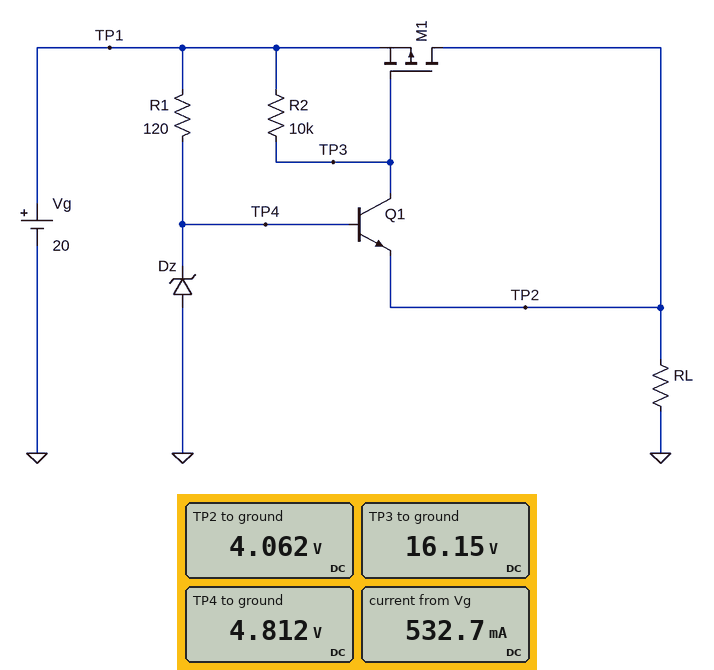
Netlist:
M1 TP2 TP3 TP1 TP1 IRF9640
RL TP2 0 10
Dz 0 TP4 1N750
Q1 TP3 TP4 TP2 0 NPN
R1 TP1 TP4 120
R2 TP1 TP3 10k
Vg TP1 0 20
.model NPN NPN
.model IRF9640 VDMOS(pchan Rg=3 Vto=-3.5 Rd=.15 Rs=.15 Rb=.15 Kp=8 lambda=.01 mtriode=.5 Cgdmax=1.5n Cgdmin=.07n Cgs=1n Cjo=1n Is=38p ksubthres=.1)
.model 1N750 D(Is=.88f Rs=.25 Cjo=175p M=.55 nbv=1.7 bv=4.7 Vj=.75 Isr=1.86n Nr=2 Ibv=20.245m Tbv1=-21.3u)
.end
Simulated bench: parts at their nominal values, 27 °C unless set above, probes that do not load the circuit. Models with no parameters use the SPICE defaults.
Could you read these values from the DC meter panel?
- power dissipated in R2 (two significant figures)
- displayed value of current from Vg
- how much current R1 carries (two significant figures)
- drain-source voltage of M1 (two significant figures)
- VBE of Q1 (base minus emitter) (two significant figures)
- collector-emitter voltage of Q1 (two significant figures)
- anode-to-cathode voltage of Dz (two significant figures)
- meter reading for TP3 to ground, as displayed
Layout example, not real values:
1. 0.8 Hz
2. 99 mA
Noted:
1. 1.5 mW
2. 532.7 mA
3. 130 mA
4. -16 V
5. 750 mV
6. 12 V
7. -4.8 V
8. 16.15 V
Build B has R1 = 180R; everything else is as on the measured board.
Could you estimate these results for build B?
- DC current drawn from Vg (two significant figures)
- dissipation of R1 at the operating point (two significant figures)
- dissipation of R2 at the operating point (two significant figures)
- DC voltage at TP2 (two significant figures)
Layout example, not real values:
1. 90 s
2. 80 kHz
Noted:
1. 490 mA
2. 1.3 W
3. 1.5 mW
4. 4.0 V
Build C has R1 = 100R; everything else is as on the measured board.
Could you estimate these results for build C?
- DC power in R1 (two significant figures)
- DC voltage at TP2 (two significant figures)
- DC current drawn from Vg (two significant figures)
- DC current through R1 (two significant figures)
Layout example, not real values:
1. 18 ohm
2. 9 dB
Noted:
1. 2.3 W
2. 4.1 V
3. 560 mA
4. 150 mA
